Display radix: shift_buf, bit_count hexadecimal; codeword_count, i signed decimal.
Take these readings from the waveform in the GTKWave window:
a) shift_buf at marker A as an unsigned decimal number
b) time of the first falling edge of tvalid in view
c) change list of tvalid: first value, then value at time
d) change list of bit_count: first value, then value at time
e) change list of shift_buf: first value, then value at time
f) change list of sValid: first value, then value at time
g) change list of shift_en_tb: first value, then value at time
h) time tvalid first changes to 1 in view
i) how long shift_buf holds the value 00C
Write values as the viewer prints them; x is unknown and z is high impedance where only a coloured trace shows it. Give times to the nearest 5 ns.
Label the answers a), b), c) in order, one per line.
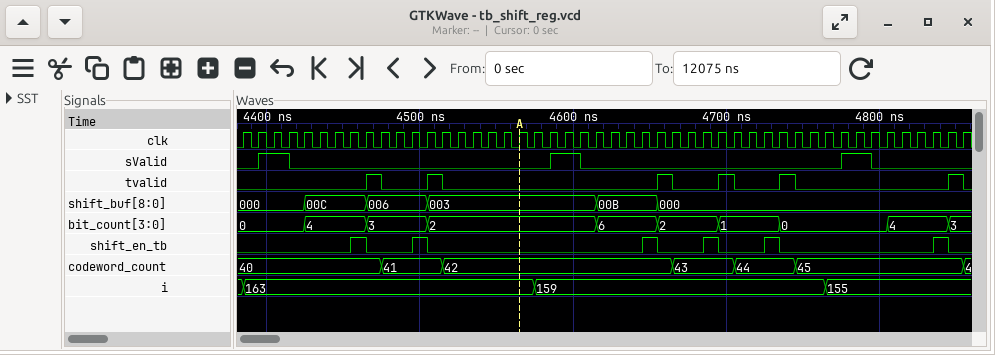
a) 3
b) 4475 ns
c) 0, 1 at 4465 ns, 0 at 4475 ns, 1 at 4505 ns, 0 at 4515 ns, 1 at 4655 ns, 0 at 4665 ns, 1 at 4695 ns, 0 at 4705 ns, 1 at 4735 ns, 0 at 4745 ns, 1 at 4845 ns, 0 at 4855 ns
d) 0, 4 at 4425 ns, 3 at 4465 ns, 2 at 4505 ns, 6 at 4615 ns, 2 at 4655 ns, 1 at 4695 ns, 0 at 4735 ns, 4 at 4805 ns, 3 at 4845 ns
e) 000, 00C at 4425 ns, 006 at 4465 ns, 003 at 4505 ns, 00B at 4615 ns, 000 at 4655 ns
f) 0, 1 at 4395 ns, 0 at 4415 ns, 1 at 4585 ns, 0 at 4605 ns, 1 at 4775 ns, 0 at 4795 ns
g) 0, 1 at 4455 ns, 0 at 4465 ns, 1 at 4495 ns, 0 at 4505 ns, 1 at 4645 ns, 0 at 4655 ns, 1 at 4685 ns, 0 at 4695 ns, 1 at 4725 ns, 0 at 4735 ns, 1 at 4835 ns, 0 at 4845 ns
h) 4465 ns
i) 40 ns
